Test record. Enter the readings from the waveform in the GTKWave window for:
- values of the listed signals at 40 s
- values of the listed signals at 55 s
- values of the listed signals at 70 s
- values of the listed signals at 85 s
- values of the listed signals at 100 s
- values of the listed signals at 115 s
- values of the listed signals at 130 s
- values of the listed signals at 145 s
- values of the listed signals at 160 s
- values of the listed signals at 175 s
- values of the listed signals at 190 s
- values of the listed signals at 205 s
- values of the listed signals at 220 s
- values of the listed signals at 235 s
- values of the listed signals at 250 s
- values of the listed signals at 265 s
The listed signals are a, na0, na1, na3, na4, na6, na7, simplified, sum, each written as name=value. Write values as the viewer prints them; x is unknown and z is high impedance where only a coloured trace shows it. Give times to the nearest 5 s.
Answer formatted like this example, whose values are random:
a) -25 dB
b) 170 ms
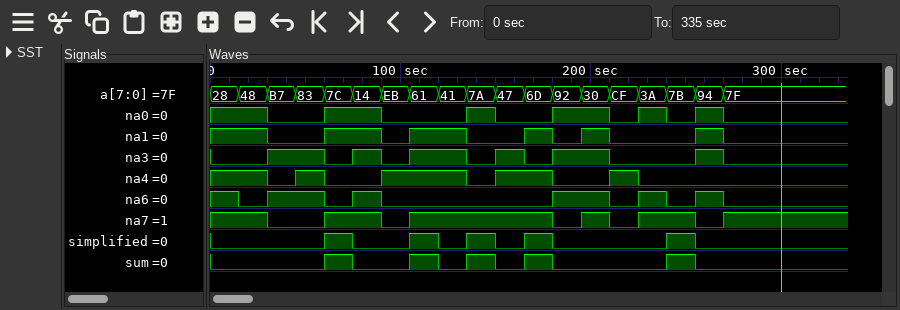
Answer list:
a) a=B7, na0=0, na1=0, na3=1, na4=0, na6=1, na7=0, simplified=0, sum=0
b) a=83, na0=0, na1=0, na3=1, na4=1, na6=1, na7=0, simplified=0, sum=0
c) a=7C, na0=1, na1=1, na3=0, na4=0, na6=0, na7=1, simplified=1, sum=1
d) a=14, na0=1, na1=1, na3=1, na4=0, na6=1, na7=1, simplified=0, sum=0
e) a=EB, na0=0, na1=0, na3=0, na4=1, na6=0, na7=0, simplified=0, sum=0
f) a=61, na0=0, na1=1, na3=1, na4=1, na6=0, na7=1, simplified=1, sum=1
g) a=41, na0=0, na1=1, na3=1, na4=1, na6=0, na7=1, simplified=0, sum=0
h) a=7A, na0=1, na1=0, na3=0, na4=0, na6=0, na7=1, simplified=1, sum=1
i) a=47, na0=0, na1=0, na3=1, na4=1, na6=0, na7=1, simplified=0, sum=0
j) a=6D, na0=0, na1=1, na3=0, na4=1, na6=0, na7=1, simplified=1, sum=1
k) a=92, na0=1, na1=0, na3=1, na4=0, na6=1, na7=0, simplified=0, sum=0
l) a=30, na0=1, na1=1, na3=1, na4=0, na6=1, na7=1, simplified=0, sum=0
m) a=CF, na0=0, na1=0, na3=0, na4=1, na6=0, na7=0, simplified=0, sum=0
n) a=3A, na0=1, na1=0, na3=0, na4=0, na6=1, na7=1, simplified=0, sum=0
o) a=7B, na0=0, na1=0, na3=0, na4=0, na6=0, na7=1, simplified=1, sum=1
p) a=94, na0=1, na1=1, na3=1, na4=0, na6=1, na7=0, simplified=0, sum=0
